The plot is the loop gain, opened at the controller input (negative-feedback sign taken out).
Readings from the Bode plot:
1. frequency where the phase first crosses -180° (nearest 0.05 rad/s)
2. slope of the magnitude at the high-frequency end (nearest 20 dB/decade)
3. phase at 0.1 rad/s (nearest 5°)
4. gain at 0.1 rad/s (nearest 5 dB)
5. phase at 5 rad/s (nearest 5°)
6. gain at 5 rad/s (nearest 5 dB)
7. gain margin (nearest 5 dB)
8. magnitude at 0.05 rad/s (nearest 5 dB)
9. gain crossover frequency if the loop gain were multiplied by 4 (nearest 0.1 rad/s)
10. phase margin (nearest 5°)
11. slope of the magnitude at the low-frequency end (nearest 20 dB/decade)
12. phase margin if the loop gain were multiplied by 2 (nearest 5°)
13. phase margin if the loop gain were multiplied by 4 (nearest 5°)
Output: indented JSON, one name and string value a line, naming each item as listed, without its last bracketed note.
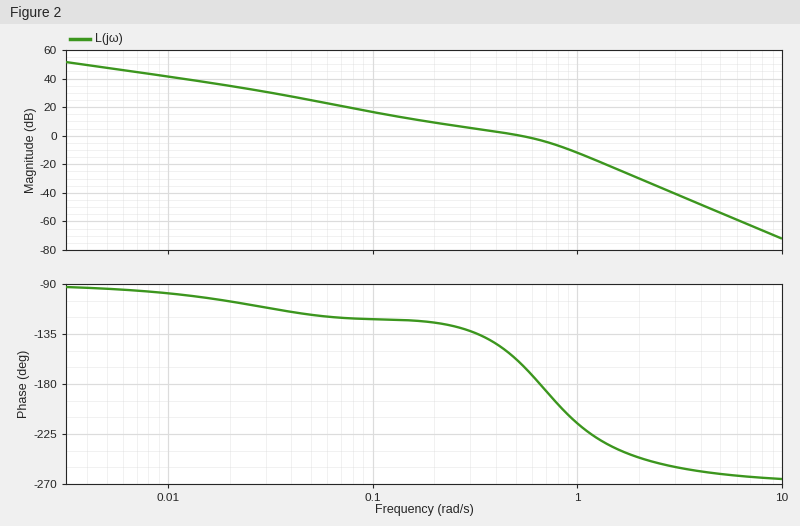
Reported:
{
  "frequency where the phase first crosses -180°": "0.65 rad/s",
  "slope of the magnitude at the high-frequency end": "-60 dB/decade",
  "phase at 0.1 rad/s": "-120°",
  "gain at 0.1 rad/s": "15 dB",
  "phase at 5 rad/s": "-260°",
  "gain at 5 rad/s": "-55 dB",
  "gain margin": "5 dB",
  "magnitude at 0.05 rad/s": "25 dB",
  "gain crossover frequency if the loop gain were multiplied by 4": "1.0 rad/s",
  "phase margin": "20°",
  "slope of the magnitude at the low-frequency end": "-20 dB/decade",
  "phase margin if the loop gain were multiplied by 2": "-15°",
  "phase margin if the loop gain were multiplied by 4": "-35°"
}
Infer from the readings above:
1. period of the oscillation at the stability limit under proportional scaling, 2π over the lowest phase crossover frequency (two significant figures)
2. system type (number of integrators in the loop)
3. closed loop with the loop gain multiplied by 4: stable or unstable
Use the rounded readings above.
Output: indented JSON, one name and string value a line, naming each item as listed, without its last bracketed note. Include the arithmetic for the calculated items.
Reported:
{
  "period of the oscillation at the stability limit under proportional scaling, 2π over the lowest phase crossover frequency": "2π / 0.65 = 9.7 s",
  "system type": "1",
  "closed loop with the loop gain multiplied by 4: stable or unstable": "unstable"
}
